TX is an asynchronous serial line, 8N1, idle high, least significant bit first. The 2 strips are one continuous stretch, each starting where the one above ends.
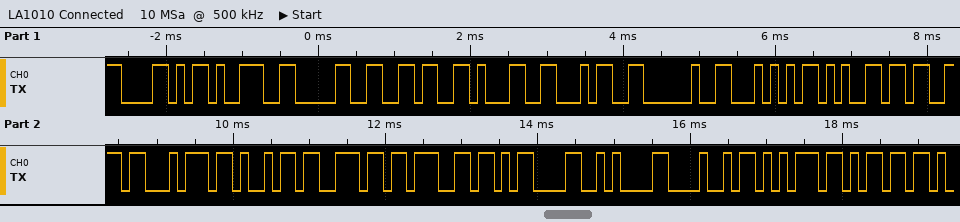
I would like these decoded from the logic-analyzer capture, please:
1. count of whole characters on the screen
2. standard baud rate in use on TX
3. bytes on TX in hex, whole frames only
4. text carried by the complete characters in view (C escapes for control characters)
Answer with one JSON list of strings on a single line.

["19", "9600 baud", "58 39 30 36 31 34 20 54 65 73 74 69 6E 67 0D 0A 48 75 6D", "\"X90614 Testing\\r\\nHum\""]
